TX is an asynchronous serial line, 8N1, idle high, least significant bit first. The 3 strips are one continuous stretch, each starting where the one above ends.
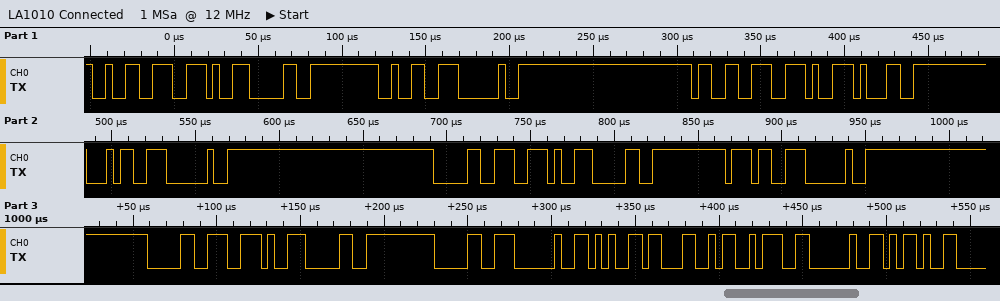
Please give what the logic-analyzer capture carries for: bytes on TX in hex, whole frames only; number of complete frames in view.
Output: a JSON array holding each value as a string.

["32 2E 30 32 20 33 2E 31 34 20 30 2E 30 37 20 30 2E 30 30 20 65 4C 3A 20 2D", "25"]
